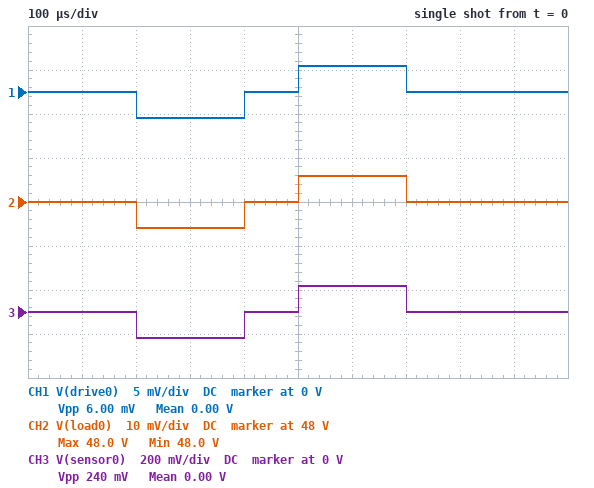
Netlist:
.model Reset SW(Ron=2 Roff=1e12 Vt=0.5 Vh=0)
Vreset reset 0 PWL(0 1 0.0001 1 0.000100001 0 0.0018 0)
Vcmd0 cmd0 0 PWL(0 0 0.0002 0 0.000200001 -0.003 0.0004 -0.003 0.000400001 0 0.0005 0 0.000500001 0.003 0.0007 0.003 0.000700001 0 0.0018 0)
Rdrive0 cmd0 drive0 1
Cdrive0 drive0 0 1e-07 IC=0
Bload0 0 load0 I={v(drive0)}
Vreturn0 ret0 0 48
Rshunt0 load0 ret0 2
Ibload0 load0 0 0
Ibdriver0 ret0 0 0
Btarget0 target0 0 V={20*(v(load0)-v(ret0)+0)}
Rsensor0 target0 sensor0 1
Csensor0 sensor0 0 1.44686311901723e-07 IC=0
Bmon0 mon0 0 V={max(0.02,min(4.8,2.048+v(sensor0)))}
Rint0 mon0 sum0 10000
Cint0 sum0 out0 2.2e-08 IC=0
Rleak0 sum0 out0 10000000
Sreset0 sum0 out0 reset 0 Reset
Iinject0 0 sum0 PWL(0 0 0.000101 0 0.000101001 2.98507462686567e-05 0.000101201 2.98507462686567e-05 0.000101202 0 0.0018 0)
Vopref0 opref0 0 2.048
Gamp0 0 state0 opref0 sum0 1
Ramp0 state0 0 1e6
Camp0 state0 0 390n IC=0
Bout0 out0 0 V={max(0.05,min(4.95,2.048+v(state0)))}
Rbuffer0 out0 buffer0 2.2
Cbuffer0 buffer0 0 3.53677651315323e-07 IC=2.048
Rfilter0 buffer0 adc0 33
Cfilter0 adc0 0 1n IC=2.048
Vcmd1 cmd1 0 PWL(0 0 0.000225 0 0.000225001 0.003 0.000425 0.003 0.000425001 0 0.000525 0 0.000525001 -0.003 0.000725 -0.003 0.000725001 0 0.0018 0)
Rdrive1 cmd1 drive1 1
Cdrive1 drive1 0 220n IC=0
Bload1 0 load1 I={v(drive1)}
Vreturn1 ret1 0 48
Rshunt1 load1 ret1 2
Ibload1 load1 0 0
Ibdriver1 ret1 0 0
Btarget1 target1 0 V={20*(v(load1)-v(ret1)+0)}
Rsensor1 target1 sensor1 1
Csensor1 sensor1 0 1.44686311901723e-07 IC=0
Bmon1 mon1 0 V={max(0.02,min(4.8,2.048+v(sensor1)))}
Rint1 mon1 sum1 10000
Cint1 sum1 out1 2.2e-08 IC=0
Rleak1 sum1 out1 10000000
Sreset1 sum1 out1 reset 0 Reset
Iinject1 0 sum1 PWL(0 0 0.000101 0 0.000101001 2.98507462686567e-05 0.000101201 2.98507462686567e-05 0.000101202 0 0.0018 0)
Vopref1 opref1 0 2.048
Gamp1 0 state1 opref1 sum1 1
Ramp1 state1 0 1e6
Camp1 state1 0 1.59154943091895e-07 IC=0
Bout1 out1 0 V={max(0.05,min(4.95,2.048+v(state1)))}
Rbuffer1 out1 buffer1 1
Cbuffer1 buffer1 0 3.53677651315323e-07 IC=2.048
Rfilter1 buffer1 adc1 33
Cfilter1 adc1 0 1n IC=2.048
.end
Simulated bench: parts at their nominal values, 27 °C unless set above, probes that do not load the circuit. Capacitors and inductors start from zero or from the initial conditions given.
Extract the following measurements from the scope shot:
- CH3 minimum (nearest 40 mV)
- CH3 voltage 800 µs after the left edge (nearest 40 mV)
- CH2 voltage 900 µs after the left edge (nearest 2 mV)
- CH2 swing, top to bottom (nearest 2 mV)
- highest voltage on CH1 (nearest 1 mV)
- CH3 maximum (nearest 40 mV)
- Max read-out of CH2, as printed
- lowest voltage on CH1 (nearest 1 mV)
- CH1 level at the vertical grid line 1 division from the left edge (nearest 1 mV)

-120 mV
0 V
48.000 V
12 mV
3 mV
120 mV
48.0 V
-3 mV
0 V
